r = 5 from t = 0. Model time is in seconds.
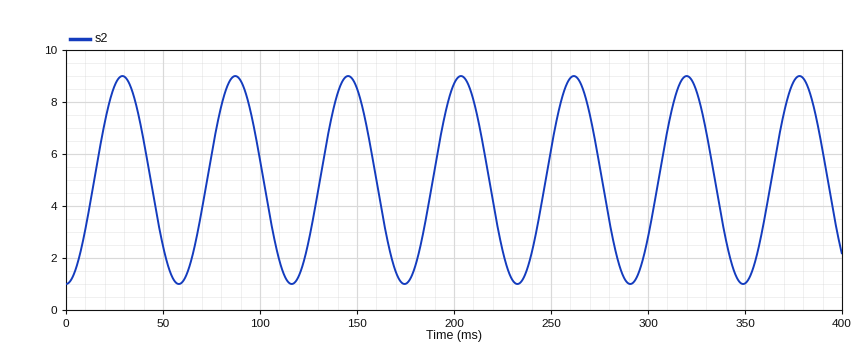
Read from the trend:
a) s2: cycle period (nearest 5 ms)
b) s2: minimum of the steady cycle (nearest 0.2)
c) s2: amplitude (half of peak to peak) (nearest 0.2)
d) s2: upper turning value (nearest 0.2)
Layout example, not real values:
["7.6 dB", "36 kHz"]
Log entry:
["60 ms", "1.0", "4.0", "9.0"]
